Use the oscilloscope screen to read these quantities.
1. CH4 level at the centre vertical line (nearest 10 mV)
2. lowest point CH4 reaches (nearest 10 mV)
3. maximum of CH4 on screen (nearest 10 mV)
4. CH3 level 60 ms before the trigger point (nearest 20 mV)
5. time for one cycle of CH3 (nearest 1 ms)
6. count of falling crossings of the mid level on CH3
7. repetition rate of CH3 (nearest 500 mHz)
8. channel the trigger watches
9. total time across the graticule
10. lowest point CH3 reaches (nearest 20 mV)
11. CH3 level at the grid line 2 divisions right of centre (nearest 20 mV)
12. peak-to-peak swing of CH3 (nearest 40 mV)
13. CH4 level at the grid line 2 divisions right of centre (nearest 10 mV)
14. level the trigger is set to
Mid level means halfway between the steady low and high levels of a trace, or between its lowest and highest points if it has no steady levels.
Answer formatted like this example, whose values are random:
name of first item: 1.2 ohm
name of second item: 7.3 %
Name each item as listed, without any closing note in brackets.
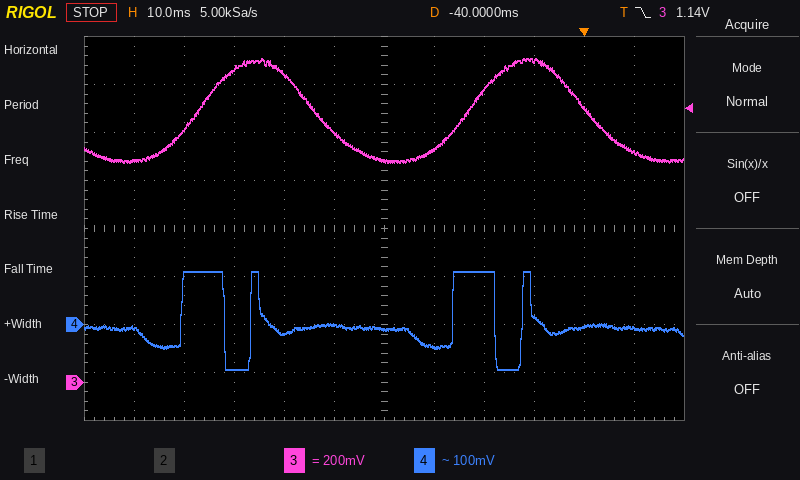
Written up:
CH4 level at the centre vertical line: -10 mV
lowest point CH4 reaches: -90 mV
maximum of CH4 on screen: 110 mV
CH3 level 60 ms before the trigger point: 1.28 V
time for one cycle of CH3: 54 ms
count of falling crossings of the mid level on CH3: 2
repetition rate of CH3: 18.5 Hz
channel the trigger watches: CH3
total time across the graticule: 120 ms
lowest point CH3 reaches: 920 mV
CH3 level at the grid line 2 divisions right of centre: 1.22 V
peak-to-peak swing of CH3: 440 mV
CH4 level at the grid line 2 divisions right of centre: 110 mV
level the trigger is set to: 1.14 V
